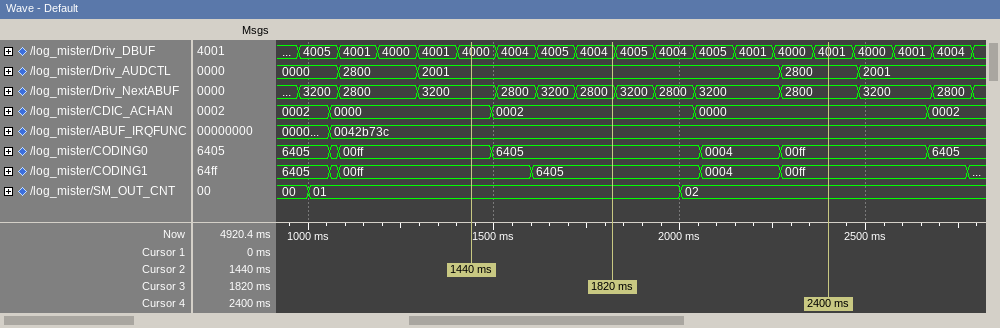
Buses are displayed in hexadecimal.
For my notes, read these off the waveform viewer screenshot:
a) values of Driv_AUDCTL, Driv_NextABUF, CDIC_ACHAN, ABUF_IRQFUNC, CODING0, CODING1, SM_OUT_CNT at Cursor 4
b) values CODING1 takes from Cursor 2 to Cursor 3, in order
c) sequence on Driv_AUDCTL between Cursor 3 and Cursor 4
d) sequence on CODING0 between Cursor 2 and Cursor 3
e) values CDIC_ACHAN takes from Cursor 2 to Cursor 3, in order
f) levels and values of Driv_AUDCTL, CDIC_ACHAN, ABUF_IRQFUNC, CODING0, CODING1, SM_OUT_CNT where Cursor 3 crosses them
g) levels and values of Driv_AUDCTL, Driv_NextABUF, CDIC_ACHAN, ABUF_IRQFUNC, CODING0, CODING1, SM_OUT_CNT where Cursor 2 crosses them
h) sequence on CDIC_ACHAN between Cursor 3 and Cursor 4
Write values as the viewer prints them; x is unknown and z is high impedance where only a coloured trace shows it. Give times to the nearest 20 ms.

Driv_AUDCTL=2800, Driv_NextABUF=2800, CDIC_ACHAN=0000, ABUF_IRQFUNC=0042b73c, CODING0=00ff, CODING1=00ff, SM_OUT_CNT=02
00ff, 6405
2001, 2800
00ff, 6405
0000, 0002
Driv_AUDCTL=2001, CDIC_ACHAN=0002, ABUF_IRQFUNC=0042b73c, CODING0=6405, CODING1=6405, SM_OUT_CNT=01
Driv_AUDCTL=2001, Driv_NextABUF=3200, CDIC_ACHAN=0000, ABUF_IRQFUNC=0042b73c, CODING0=00ff, CODING1=00ff, SM_OUT_CNT=01
0002, 0000
